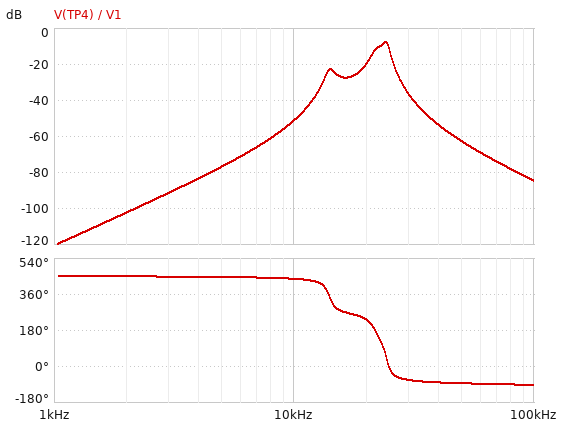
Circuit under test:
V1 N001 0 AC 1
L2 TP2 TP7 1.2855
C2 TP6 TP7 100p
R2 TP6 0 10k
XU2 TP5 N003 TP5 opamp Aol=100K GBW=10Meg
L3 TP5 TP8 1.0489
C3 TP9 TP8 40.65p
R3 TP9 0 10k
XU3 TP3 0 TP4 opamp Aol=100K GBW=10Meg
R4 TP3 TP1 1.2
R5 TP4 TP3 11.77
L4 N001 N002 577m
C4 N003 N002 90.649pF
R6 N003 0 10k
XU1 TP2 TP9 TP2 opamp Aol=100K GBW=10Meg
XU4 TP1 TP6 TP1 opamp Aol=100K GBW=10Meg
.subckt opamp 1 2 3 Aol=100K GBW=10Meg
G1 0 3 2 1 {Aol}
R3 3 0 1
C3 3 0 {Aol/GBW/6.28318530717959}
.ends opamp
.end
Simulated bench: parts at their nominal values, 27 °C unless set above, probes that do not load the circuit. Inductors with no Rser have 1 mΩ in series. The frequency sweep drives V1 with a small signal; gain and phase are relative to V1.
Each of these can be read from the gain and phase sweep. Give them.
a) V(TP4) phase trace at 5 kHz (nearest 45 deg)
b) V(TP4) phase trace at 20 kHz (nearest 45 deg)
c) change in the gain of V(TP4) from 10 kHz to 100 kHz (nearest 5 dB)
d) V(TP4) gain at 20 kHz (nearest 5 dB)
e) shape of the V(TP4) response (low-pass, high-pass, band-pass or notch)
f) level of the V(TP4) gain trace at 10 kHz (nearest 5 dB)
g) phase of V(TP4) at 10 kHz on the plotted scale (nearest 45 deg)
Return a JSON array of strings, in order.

["450 deg", "225 deg", "-35 dB", "-20 dB", "band-pass", "-50 dB", "450 deg"]
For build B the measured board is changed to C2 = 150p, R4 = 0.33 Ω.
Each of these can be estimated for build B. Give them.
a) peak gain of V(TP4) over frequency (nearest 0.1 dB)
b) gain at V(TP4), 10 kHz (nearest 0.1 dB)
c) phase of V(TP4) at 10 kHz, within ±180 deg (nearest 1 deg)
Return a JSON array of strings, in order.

["2.0 dB", "-30.8 dB", "60 deg"]
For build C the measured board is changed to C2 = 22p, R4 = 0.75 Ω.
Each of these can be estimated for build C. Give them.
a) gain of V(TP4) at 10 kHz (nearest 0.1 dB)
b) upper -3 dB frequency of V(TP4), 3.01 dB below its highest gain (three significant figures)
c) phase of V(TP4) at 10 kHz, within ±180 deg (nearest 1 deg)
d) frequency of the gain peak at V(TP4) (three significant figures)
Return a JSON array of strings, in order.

["-65.4 dB", "25.1 kHz", "82 deg", "24.3 kHz"]
